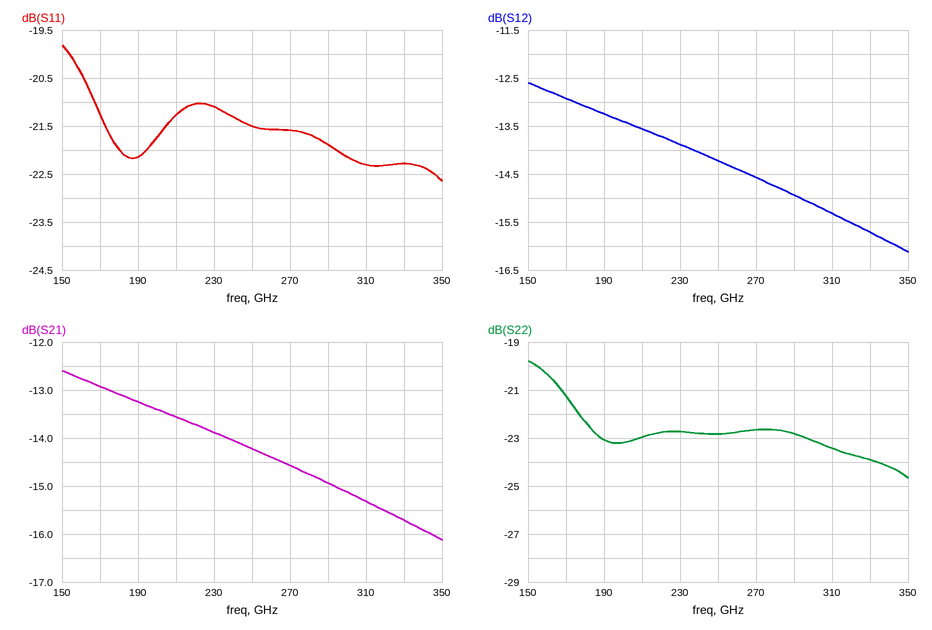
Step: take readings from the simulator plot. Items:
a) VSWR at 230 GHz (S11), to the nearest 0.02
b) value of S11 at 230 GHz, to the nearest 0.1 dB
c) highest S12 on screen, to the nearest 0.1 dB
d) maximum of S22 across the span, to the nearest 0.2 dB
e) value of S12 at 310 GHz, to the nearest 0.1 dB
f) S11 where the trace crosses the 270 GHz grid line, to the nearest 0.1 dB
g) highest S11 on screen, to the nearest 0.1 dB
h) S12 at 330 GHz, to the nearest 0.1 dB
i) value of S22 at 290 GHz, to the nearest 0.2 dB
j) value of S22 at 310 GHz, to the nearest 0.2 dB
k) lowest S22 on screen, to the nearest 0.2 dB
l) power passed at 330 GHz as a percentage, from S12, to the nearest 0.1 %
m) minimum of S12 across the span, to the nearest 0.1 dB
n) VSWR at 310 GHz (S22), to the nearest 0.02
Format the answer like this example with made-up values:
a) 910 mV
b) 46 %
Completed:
a) 1.20
b) -21.1 dB
c) -12.6 dB
d) -19.8 dB
e) -15.3 dB
f) -21.6 dB
g) -19.8 dB
h) -15.7 dB
i) -22.8 dB
j) -23.4 dB
k) -24.6 dB
l) 2.7 %
m) -16.1 dB
n) 1.14
